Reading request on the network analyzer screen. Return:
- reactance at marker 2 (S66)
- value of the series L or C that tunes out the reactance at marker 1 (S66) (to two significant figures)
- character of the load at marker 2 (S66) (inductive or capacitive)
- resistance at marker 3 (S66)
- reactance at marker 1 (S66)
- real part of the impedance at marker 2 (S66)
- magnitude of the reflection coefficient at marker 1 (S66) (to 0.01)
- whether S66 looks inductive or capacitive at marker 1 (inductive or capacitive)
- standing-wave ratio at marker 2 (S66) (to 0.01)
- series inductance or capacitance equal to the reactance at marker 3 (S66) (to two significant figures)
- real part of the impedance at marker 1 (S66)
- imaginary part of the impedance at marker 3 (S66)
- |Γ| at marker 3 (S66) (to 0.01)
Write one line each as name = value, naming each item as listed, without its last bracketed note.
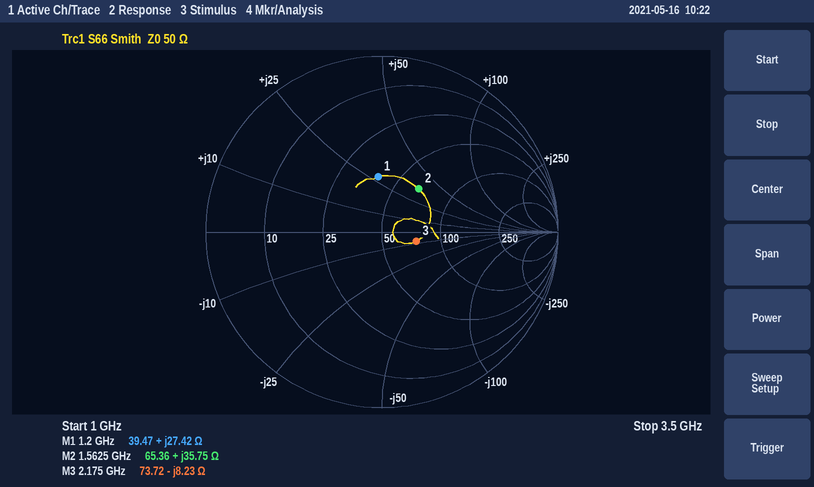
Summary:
reactance at marker 2 = +35.75 Ω
value of the series L or C that tunes out the reactance at marker 1 (S66) = 4.8 pF
character of the load at marker 2 (S66) = inductive
resistance at marker 3 = 73.72 Ω
reactance at marker 1 = +27.42 Ω
real part of the impedance at marker 2 = 65.36 Ω
magnitude of the reflection coefficient at marker 1 (S66) = 0.31
whether S66 looks inductive or capacitive at marker 1 = inductive
standing-wave ratio at marker 2 (S66) = 1.95
series inductance or capacitance equal to the reactance at marker 3 (S66) = 8.9 pF
real part of the impedance at marker 1 = 39.47 Ω
imaginary part of the impedance at marker 3 = -8.23 Ω
|Γ| at marker 3 (S66) = 0.20
